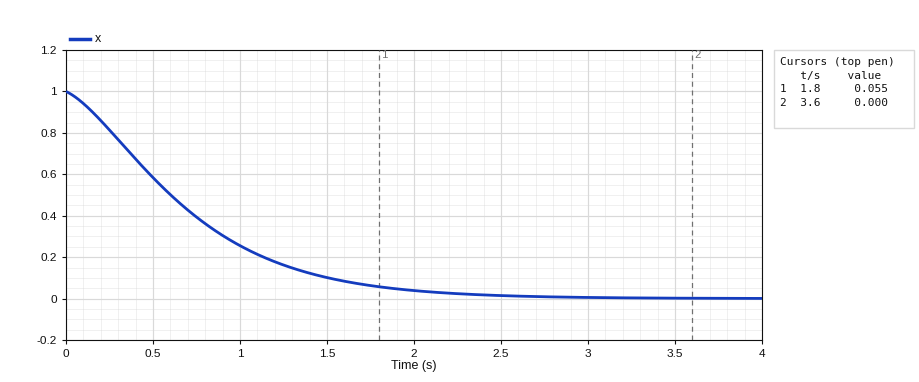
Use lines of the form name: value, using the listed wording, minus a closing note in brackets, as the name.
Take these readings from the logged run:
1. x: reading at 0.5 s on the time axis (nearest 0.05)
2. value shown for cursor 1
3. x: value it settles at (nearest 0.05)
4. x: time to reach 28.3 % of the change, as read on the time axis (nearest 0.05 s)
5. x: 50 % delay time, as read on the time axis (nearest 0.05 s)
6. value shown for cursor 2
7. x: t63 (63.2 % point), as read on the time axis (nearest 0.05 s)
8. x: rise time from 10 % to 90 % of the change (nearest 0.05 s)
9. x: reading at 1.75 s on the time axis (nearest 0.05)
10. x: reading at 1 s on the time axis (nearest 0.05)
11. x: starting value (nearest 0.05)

x: reading at 0.5 s on the time axis: 0.60
value shown for cursor 1: 0.055
x: value it settles at: 0.00
x: time to reach 28.3 % of the change, as read on the time axis: 0.35 s
x: 50 % delay time, as read on the time axis: 0.60 s
value shown for cursor 2: 0.000
x: t63 (63.2 % point), as read on the time axis: 0.80 s
x: rise time from 10 % to 90 % of the change: 1.35 s
x: reading at 1.75 s on the time axis: 0.05
x: reading at 1 s on the time axis: 0.25
x: starting value: 1.00
